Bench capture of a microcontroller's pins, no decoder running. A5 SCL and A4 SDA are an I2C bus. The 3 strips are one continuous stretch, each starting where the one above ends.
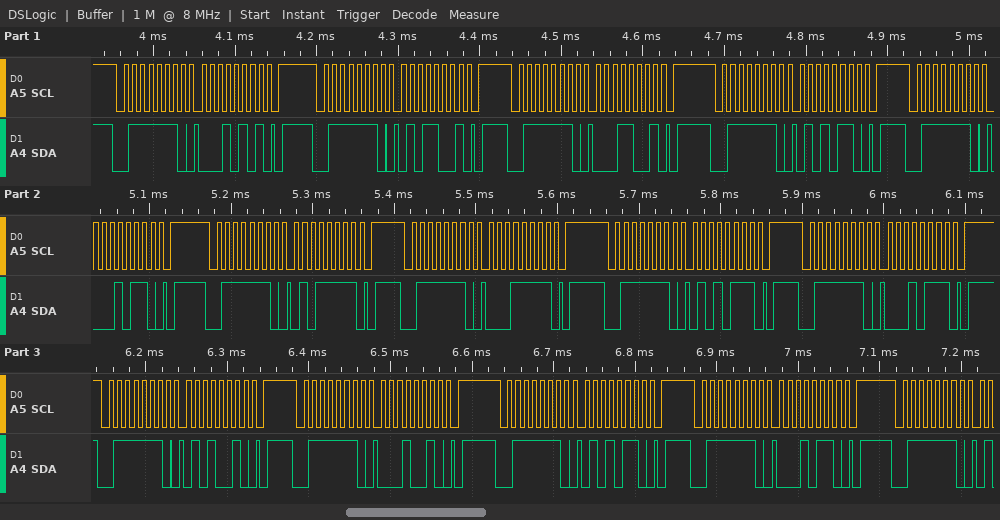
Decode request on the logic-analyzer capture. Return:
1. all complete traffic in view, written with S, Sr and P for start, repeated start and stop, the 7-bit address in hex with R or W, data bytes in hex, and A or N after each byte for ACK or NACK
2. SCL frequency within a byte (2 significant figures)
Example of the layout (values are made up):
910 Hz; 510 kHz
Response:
S 3FW A 15 A P S 3FW A 59 A P S 3FW A 19 A P S 3FW A 56 A P S 3FW A 16 A P S 3FW A 5F A P S 3FW A 1F A P S 3FW A 57 A P S 3FW A 17 A P S 3FW A 52 A P S 3FW A 12 A P S 3FW A 56 A P S 3FW A 16 A P S 3FW A; 100 kHz
